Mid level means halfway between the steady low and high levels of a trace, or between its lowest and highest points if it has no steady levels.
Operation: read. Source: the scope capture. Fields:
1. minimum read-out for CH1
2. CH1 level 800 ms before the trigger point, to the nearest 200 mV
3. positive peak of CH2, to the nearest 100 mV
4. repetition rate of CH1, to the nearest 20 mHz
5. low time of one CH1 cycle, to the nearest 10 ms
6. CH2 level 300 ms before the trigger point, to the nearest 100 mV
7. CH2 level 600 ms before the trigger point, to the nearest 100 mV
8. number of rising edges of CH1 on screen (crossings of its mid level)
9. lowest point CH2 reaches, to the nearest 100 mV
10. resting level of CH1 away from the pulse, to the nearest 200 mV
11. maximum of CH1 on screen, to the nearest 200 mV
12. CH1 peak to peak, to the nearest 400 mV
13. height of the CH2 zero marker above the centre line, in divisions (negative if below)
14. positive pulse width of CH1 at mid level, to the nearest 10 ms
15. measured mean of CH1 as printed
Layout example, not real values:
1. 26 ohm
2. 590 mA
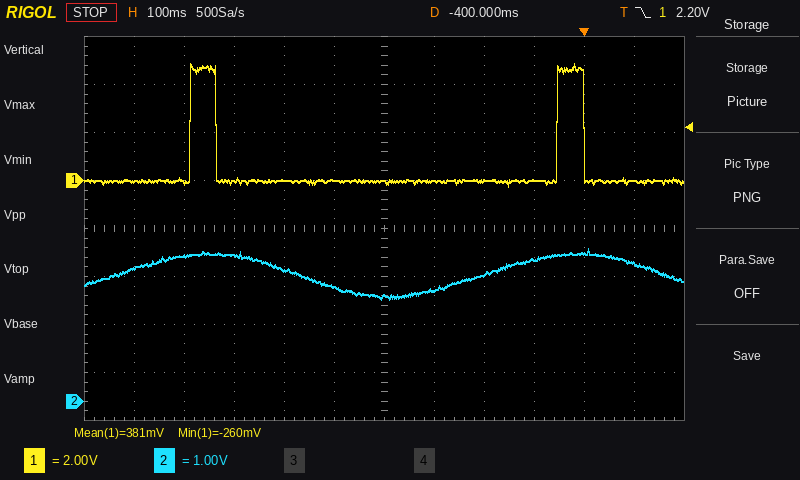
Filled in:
1. -260 mV
2. 0.0 V
3. 3.2 V
4. 1.36 Hz
5. 680 ms
6. 2.3 V
7. 2.7 V
8. 2
9. 2.1 V
10. 0.0 V
11. 4.8 V
12. 5.2 V
13. -3.6 div
14. 50 ms
15. 381 mV
